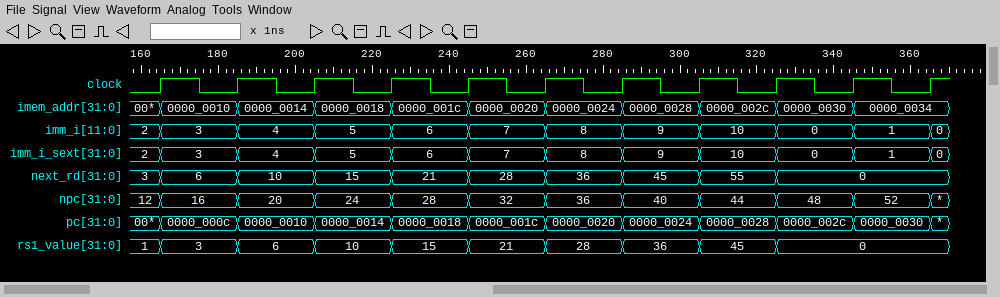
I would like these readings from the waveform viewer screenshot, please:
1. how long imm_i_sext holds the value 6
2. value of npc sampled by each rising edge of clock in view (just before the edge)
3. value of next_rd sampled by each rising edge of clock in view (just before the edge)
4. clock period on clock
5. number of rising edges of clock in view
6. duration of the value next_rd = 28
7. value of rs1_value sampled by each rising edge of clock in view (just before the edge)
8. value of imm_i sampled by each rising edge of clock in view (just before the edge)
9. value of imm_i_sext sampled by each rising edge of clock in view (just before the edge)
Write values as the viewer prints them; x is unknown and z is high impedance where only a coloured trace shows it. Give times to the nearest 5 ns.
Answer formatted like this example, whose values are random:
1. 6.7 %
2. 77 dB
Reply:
1. 20 ns
2. 12, 16, 20, 24, 28, 32, 36, 40, 44, 48, 52
3. 3, 6, 10, 15, 21, 28, 36, 45, 55, 0, 0
4. 20 ns
5. 11
6. 20 ns
7. 1, 3, 6, 10, 15, 21, 28, 36, 45, 0, 0
8. 2, 3, 4, 5, 6, 7, 8, 9, 10, 0, 1
9. 2, 3, 4, 5, 6, 7, 8, 9, 10, 0, 1
